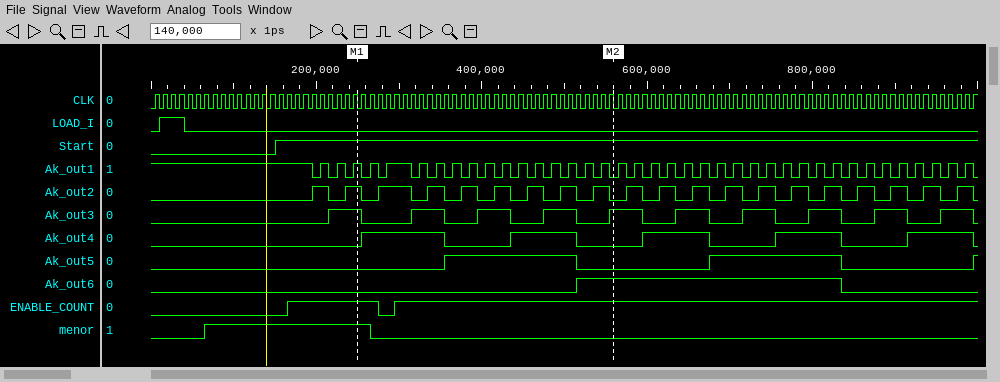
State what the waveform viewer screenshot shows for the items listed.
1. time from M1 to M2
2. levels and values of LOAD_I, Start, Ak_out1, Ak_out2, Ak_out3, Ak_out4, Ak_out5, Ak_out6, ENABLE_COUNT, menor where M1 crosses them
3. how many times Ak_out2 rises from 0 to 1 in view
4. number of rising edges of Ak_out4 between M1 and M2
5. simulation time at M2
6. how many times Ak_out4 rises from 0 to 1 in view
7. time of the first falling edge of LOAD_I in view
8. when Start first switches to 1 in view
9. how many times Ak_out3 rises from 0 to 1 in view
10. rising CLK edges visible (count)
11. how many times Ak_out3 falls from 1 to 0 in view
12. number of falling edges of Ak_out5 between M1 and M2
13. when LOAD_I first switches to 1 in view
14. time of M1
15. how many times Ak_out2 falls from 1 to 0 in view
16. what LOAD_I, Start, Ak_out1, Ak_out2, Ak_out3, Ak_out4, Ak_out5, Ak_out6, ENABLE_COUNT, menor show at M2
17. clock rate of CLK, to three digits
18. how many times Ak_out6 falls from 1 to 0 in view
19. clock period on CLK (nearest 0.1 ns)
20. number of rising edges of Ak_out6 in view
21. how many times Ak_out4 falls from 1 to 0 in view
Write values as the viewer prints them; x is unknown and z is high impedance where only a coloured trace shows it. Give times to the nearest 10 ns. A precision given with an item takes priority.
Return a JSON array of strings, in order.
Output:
["310 ns", "LOAD_I=0, Start=1, Ak_out1=1, Ak_out2=1, Ak_out3=1, Ak_out4=0, Ak_out5=0, Ak_out6=0, ENABLE_COUNT=1, menor=1", "20", "2", "560 ns", "5", "40 ns", "150 ns", "10", "100", "10", "1", "10 ns", "250 ns", "20", "LOAD_I=0, Start=1, Ak_out1=0, Ak_out2=0, Ak_out3=1, Ak_out4=0, Ak_out5=0, Ak_out6=1, ENABLE_COUNT=1, menor=0", "100 MHz", "1", "10 ns", "1", "5"]
